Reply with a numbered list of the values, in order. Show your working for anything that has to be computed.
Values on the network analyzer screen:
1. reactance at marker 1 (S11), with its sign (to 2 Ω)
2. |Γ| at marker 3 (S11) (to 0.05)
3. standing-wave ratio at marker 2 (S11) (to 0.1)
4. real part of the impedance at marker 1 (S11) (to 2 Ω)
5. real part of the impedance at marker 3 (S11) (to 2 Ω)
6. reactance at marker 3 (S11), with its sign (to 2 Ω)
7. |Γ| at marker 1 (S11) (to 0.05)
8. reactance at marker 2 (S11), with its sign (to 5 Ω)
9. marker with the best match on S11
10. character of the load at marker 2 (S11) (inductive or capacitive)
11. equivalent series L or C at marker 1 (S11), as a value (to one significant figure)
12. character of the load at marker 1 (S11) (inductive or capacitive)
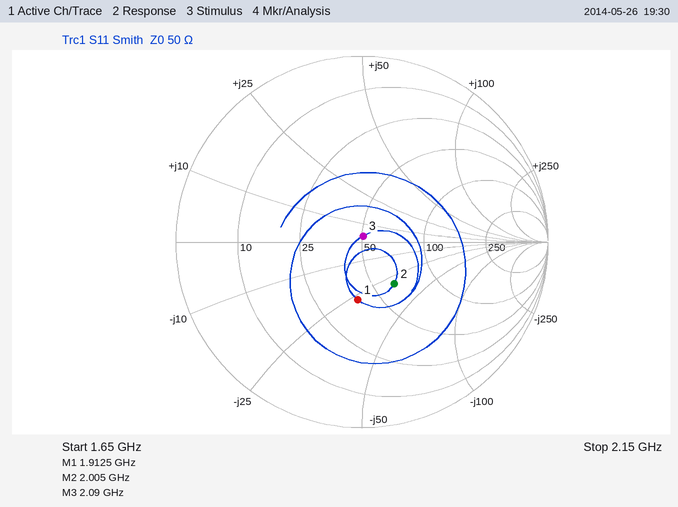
1. -28 Ω
2. 0.05
3. 1.8
4. 40 Ω
5. 50 Ω
6. +4 Ω
7. 0.30
8. -30 Ω
9. marker 3
10. capacitive
11. C = 1/(2π × 1.9125 GHz × 28 Ω) ≈ 3 pF
12. capacitive
